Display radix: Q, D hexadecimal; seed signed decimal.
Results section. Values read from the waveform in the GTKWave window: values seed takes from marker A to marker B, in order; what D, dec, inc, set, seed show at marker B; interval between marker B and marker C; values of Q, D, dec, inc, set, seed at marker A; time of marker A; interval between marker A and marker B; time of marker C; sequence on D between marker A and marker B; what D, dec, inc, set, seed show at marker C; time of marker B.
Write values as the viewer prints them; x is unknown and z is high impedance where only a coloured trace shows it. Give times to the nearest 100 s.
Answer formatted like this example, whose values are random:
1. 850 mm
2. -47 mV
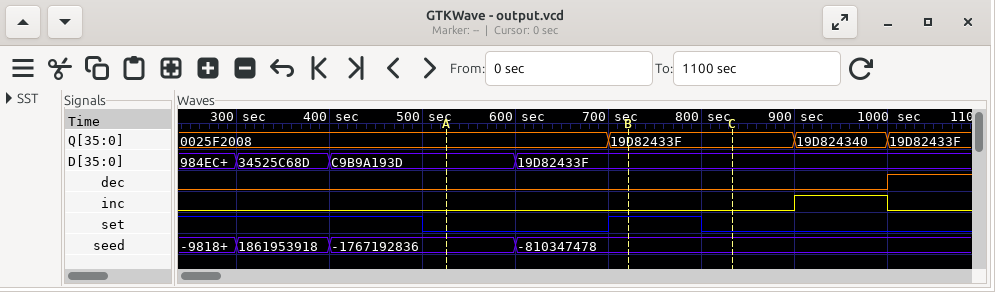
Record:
1. -1767192836, -810347478
2. D=19D82433F, dec=0, inc=0, set=1, seed=-810347478
3. 100 s
4. Q=0025F2008, D=C9B9A193D, dec=0, inc=0, set=0, seed=-1767192836
5. 500 s
6. 200 s
7. 800 s
8. C9B9A193D, 19D82433F
9. D=19D82433F, dec=0, inc=0, set=0, seed=-810347478
10. 700 s
